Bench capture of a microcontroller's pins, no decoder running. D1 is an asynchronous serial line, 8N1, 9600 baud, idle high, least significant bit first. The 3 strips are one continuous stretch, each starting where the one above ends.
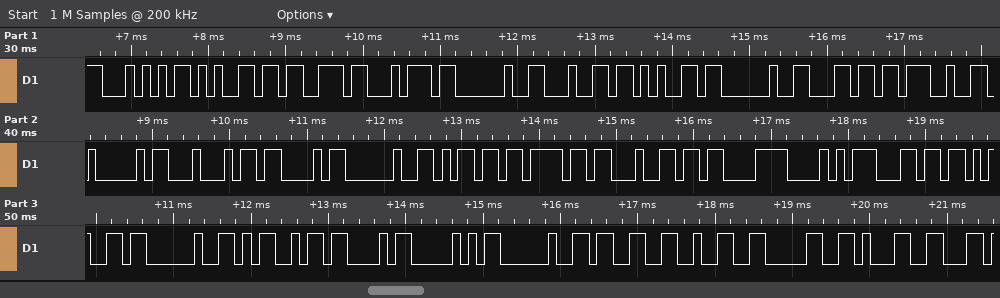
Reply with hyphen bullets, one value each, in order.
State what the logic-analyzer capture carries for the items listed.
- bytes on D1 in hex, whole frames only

- 54 65 73 74 20 64 65 20 6C 27 41 44 43 20 6D 6F 64 C3 A8 6C 65 20 4D 43 50 20 33 32 30 31
